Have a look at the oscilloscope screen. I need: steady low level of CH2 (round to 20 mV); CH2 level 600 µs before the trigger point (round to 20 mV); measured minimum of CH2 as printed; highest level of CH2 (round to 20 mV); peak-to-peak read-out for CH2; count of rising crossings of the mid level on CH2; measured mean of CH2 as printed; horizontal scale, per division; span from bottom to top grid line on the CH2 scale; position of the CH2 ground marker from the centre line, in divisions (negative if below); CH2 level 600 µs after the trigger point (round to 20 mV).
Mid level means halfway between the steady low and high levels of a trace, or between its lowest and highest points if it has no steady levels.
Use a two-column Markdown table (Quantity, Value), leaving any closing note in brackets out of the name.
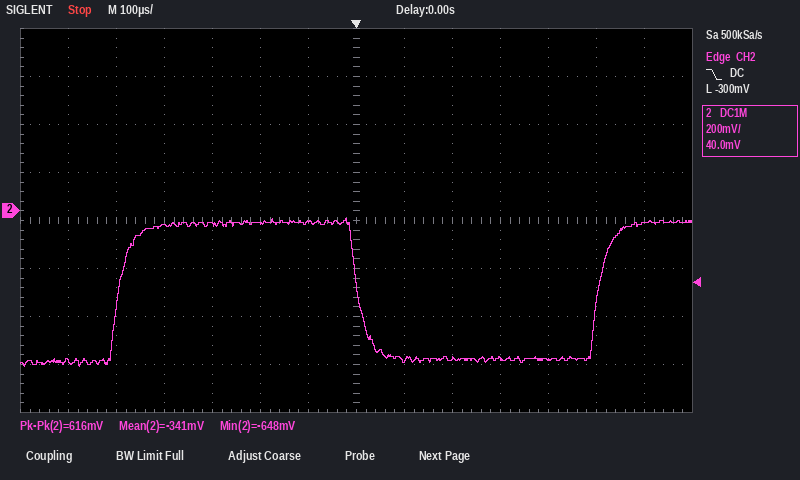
| Quantity | Value |
|---|---|
| steady low level of CH2 | -620 mV |
| CH2 level 600 µs before the trigger point | -620 mV |
| measured minimum of CH2 as printed | -648 mV |
| highest level of CH2 | -40 mV |
| peak-to-peak read-out for CH2 | 616 mV |
| count of rising crossings of the mid level on CH2 | 2 |
| measured mean of CH2 as printed | -341 mV |
| horizontal scale, per division | 100 µs |
| span from bottom to top grid line on the CH2 scale | 1.6 V |
| position of the CH2 ground marker from the centre line, in divisions | +0.2 div |
| CH2 level 600 µs after the trigger point | -40 mV |
